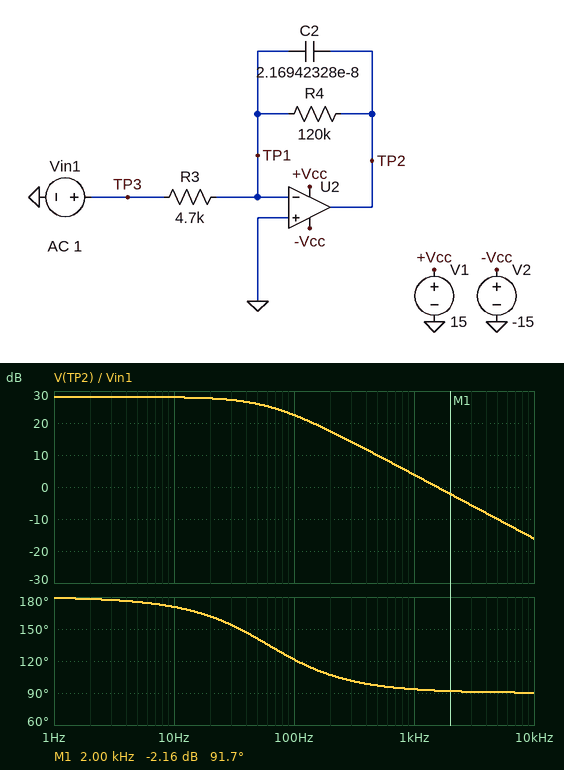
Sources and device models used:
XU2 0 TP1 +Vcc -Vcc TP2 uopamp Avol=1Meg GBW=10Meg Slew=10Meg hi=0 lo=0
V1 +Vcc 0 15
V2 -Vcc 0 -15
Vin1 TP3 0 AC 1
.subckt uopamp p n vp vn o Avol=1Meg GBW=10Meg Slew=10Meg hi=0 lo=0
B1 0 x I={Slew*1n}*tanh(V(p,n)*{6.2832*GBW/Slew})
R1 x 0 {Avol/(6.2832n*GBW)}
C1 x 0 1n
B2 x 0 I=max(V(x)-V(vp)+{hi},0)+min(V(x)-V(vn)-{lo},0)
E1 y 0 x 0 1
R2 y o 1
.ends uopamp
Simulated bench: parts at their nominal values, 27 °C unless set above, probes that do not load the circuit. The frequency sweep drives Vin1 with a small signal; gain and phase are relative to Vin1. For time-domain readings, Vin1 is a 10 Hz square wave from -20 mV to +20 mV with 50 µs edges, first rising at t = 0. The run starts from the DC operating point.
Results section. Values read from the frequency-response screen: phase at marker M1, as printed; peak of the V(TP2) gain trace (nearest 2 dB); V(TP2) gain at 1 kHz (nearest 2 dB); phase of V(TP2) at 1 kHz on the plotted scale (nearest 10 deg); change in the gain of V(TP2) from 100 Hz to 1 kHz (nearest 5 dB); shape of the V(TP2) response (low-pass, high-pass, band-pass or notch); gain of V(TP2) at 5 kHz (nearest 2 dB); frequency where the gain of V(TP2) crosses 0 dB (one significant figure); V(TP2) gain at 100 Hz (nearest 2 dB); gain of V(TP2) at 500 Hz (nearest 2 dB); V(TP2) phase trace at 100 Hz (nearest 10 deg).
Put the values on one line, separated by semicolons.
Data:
91.7 deg; 28 dB; 4 dB; 90 deg; -20 dB; low-pass; -10 dB; 2 kHz; 22 dB; 10 dB; 120 deg
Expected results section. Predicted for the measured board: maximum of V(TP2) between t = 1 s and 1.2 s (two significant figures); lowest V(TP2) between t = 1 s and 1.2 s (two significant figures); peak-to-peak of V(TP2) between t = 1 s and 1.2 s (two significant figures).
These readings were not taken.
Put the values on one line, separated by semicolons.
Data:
510 mV; -510 mV; 1.0 V
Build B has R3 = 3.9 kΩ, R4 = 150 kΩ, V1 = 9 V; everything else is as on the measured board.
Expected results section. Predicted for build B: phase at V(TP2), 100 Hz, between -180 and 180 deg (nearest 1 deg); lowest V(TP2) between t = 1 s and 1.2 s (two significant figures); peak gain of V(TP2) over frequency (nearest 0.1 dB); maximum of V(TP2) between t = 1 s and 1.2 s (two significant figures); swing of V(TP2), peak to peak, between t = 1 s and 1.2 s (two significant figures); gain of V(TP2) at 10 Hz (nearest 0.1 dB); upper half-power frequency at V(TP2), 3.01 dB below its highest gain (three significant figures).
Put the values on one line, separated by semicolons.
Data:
116 deg; -770 mV; 31.7 dB; 770 mV; 1.5 V; 31.5 dB; 48.9 Hz
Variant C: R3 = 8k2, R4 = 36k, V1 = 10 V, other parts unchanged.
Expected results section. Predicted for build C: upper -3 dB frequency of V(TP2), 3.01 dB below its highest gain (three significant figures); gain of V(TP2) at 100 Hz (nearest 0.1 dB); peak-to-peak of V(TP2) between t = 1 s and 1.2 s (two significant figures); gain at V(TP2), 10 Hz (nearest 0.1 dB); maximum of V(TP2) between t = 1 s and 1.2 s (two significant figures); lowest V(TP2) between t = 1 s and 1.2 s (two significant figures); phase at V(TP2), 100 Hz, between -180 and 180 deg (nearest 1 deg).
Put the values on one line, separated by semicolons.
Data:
204 Hz; 11.9 dB; 180 mV; 12.8 dB; 88 mV; -88 mV; 154 deg
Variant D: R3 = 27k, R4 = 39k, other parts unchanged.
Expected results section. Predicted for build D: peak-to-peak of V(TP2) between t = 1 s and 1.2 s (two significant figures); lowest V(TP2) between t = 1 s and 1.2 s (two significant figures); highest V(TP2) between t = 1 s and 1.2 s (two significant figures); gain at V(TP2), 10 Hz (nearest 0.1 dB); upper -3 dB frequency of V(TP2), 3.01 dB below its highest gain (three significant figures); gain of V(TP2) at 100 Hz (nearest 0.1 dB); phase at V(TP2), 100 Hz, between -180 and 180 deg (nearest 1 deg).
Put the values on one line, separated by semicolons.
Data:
58 mV; -29 mV; 29 mV; 3.2 dB; 188 Hz; 2.1 dB; 152 deg
